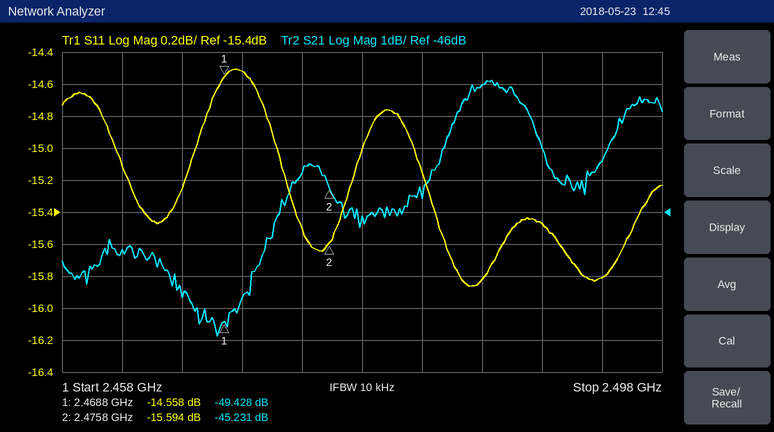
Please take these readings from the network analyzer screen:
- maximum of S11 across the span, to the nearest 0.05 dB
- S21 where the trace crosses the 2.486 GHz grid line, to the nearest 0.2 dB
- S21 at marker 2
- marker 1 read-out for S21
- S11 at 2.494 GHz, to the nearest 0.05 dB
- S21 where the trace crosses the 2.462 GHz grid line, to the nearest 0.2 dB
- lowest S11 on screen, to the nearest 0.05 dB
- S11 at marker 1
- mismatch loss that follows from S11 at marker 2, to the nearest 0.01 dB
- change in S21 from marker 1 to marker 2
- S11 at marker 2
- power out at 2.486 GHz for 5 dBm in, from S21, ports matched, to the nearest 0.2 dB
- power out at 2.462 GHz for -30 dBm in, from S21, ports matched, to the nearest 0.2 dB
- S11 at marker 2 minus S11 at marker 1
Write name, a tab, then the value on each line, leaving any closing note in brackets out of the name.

maximum of S11 across the span, to the nearest 0.05 dB	-14.50 dB
S21 where the trace crosses the 2.486 GHz grid line, to the nearest 0.2 dB	-42.0 dB
S21 at marker 2	-45.231 dB
marker 1 read-out for S21	-49.428 dB
S11 at 2.494 GHz, to the nearest 0.05 dB	-15.80 dB
S21 where the trace crosses the 2.462 GHz grid line, to the nearest 0.2 dB	-47.2 dB
lowest S11 on screen, to the nearest 0.05 dB	-15.85 dB
S11 at marker 1	-14.558 dB
mismatch loss that follows from S11 at marker 2, to the nearest 0.01 dB	0.12 dB
change in S21 from marker 1 to marker 2	4.197 dB
S11 at marker 2	-15.594 dB
power out at 2.486 GHz for 5 dBm in, from S21, ports matched, to the nearest 0.2 dB	-37.0 dBm
power out at 2.462 GHz for -30 dBm in, from S21, ports matched, to the nearest 0.2 dB	-77.2 dBm
S11 at marker 2 minus S11 at marker 1	-1.036 dB
